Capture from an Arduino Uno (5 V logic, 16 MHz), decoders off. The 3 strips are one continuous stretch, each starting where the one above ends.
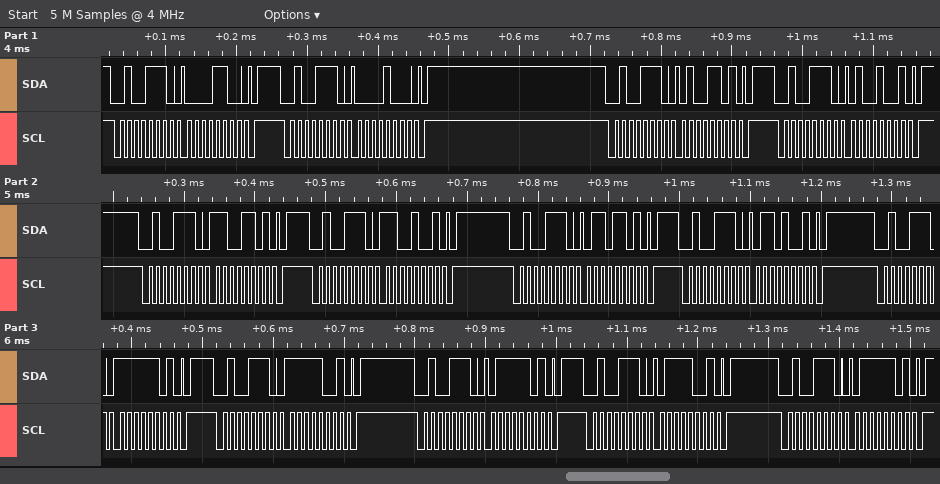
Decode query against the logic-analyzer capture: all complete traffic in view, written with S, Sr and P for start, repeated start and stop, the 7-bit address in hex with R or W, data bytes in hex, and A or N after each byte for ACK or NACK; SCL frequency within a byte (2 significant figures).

S 27W A 0C A P S 27W A 08 A P S 27W A 4D A P S 27W A 49 A P S 27W A CD A P S 27W A C9 A P S 27W A 6D A P S 27W A 69 A P S 27W A FD A P S 27W A F9 A P S 27W A 7D A P S 27W A 79 A P S 27W A 7D A P
100 kHz
